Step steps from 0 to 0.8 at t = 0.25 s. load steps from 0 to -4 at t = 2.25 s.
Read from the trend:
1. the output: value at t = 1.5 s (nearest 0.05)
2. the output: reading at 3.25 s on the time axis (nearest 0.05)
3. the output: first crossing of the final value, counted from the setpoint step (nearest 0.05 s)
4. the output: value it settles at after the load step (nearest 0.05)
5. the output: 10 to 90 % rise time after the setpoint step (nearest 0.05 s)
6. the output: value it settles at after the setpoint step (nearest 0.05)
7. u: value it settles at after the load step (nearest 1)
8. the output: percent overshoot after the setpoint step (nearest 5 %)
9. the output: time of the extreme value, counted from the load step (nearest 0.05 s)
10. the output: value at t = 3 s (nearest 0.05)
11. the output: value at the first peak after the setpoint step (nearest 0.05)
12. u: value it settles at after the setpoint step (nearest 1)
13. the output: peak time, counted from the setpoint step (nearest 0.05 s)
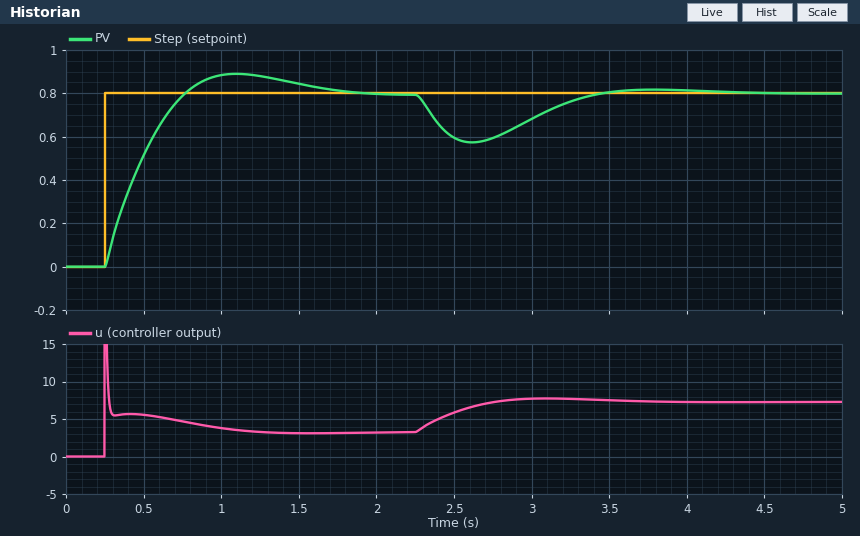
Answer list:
0.85
0.75
0.50 s
0.80
0.40 s
0.80
7
10 %
0.35 s
0.70
0.90
3
0.85 s
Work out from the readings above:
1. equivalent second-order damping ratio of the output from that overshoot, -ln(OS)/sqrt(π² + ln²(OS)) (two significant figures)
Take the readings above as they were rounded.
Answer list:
0.59
